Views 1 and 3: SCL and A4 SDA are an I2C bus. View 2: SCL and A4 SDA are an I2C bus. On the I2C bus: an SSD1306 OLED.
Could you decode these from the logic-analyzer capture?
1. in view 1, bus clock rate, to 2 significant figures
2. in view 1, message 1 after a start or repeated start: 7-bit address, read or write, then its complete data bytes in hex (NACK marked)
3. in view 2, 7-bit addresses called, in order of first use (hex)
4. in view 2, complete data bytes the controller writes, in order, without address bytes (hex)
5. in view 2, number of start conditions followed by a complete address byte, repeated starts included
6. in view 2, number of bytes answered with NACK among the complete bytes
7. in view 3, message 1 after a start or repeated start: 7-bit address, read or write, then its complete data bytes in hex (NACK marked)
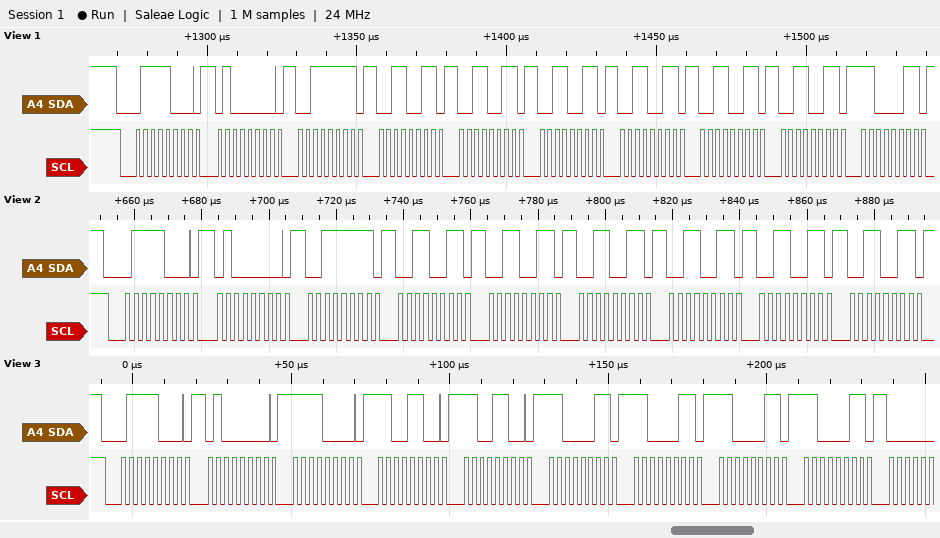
400 kHz
0x3C write: 40 3F 33 33 33 33 33 33 C3
0x3C
40 3F 33 33 33 33 33 33
1
0
0x3C write: 40 F0 CC CC C3 C3 C3 C3
